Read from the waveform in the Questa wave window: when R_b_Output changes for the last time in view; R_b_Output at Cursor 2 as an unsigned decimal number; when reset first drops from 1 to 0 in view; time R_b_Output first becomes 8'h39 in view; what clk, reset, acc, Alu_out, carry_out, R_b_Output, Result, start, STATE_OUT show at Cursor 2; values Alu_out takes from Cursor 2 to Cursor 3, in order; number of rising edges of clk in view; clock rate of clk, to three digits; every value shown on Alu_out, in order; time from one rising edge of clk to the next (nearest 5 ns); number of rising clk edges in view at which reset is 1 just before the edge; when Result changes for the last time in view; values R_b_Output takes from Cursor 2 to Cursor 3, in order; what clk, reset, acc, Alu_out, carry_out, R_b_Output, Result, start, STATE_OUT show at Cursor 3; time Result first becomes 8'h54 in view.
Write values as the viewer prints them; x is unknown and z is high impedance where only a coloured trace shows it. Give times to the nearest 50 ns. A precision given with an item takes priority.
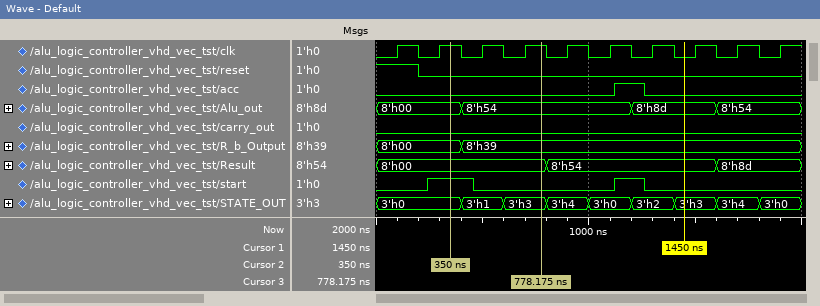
400 ns
0
200 ns
400 ns
clk=1, reset=0, acc=0, Alu_out=8'h00, carry_out=0, R_b_Output=8'h00, Result=8'h00, start=1, STATE_OUT=3'h0
8'h00, 8'h54
10
5.00 MHz
8'h00, 8'h54, 8'h8d, 8'h54
200 ns
1
1600 ns
8'h00, 8'h39
clk=1, reset=0, acc=0, Alu_out=8'h54, carry_out=0, R_b_Output=8'h39, Result=8'h00, start=0, STATE_OUT=3'h3
800 ns
